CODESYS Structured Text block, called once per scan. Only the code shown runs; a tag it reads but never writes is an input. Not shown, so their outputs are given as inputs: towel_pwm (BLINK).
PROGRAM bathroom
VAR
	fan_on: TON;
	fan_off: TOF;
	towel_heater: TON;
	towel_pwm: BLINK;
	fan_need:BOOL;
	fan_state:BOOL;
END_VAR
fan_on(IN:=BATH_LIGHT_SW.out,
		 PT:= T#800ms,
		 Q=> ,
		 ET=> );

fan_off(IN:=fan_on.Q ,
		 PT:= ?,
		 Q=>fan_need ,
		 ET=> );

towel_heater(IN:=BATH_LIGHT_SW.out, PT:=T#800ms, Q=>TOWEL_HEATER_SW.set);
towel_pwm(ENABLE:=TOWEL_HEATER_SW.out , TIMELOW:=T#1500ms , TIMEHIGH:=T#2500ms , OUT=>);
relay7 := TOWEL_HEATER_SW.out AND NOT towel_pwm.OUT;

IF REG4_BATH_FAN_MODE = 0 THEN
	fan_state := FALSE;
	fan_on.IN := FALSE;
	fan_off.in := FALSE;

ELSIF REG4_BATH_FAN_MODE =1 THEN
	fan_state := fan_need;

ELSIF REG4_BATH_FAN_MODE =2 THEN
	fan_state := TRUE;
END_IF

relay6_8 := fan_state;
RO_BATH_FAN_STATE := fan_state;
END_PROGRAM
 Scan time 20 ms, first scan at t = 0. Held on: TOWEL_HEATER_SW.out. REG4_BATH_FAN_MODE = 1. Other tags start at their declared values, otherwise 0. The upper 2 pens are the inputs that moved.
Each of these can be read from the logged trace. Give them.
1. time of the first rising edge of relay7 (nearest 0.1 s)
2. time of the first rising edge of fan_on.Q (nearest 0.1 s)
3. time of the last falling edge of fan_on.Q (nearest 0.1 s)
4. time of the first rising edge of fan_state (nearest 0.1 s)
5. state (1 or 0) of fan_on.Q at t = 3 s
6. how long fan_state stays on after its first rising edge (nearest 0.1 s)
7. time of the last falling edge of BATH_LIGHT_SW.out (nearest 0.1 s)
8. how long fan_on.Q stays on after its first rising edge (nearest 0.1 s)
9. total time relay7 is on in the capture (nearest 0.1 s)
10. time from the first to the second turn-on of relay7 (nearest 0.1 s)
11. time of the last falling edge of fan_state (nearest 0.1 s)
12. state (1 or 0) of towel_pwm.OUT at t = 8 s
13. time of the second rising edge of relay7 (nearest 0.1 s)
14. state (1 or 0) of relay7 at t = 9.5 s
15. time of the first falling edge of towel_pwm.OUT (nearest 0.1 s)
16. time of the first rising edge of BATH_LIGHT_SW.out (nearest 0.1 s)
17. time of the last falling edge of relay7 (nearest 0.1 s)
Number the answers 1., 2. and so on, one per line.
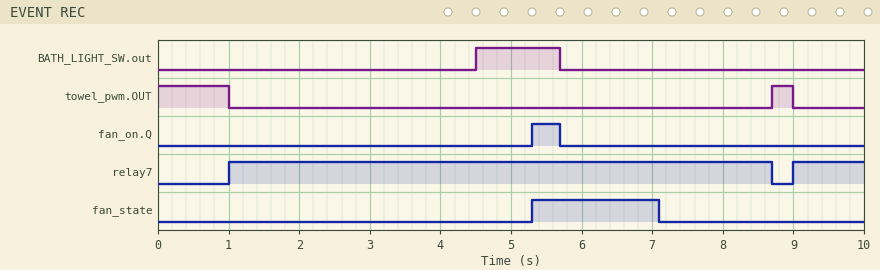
1. 1.0 s
2. 5.3 s
3. 5.7 s
4. 5.3 s
5. 0
6. 1.8 s
7. 5.7 s
8. 0.4 s
9. 8.7 s
10. 8.0 s
11. 7.1 s
12. 0
13. 9.0 s
14. 1
15. 1.0 s
16. 4.5 s
17. 8.7 s
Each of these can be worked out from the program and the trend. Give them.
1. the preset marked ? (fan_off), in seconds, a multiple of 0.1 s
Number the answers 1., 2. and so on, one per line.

1. 1.4 s
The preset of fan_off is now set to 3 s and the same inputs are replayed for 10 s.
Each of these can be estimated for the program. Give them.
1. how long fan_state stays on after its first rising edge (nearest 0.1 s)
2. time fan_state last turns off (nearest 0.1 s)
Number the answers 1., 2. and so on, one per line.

1. 3.4 s
2. 8.7 s
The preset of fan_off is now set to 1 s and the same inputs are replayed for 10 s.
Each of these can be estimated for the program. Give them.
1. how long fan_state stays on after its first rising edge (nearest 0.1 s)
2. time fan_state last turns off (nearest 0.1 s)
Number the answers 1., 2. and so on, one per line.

1. 1.4 s
2. 6.7 s
